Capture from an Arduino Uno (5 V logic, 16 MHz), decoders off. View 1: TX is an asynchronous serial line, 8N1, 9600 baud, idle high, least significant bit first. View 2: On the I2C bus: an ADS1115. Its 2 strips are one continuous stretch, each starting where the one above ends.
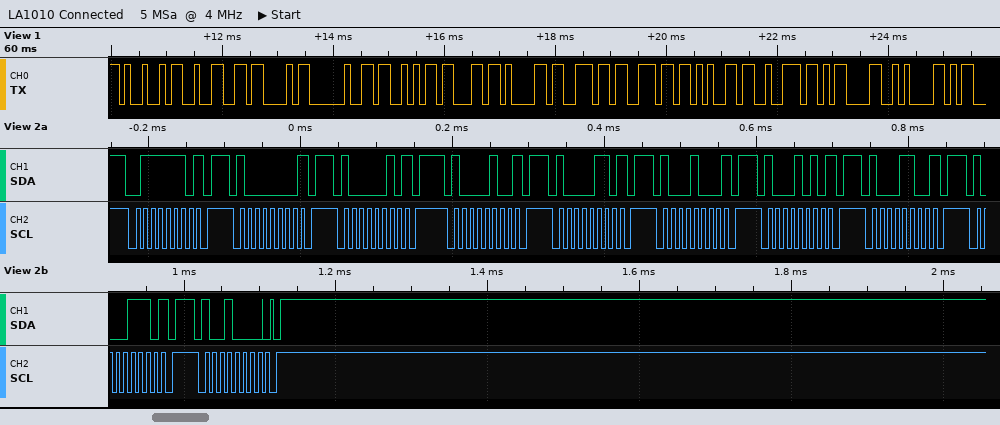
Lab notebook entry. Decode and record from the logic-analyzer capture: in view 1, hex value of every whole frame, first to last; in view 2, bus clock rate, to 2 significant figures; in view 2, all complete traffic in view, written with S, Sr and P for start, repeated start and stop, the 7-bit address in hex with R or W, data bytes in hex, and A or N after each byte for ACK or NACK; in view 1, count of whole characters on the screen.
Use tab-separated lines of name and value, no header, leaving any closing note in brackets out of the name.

in view 1, hex value of every whole frame, first to last	49 32 43 20 53 63 61 6E 6E 65 72 0D 0A
in view 2, bus clock rate, to 2 significant figures	100 kHz
in view 2, all complete traffic in view, written with S, Sr and P for start, repeated start and stop, the 7-bit address in hex with R or W, data bytes in hex, and A or N after each byte for ACK or NACK	S 3FW N P S 40W N P S 41W N P S 42W N P S 43W N P S 44W N P S 45W N P S 46W N P S 47W N P S 48W A P
in view 1, count of whole characters on the screen	13
